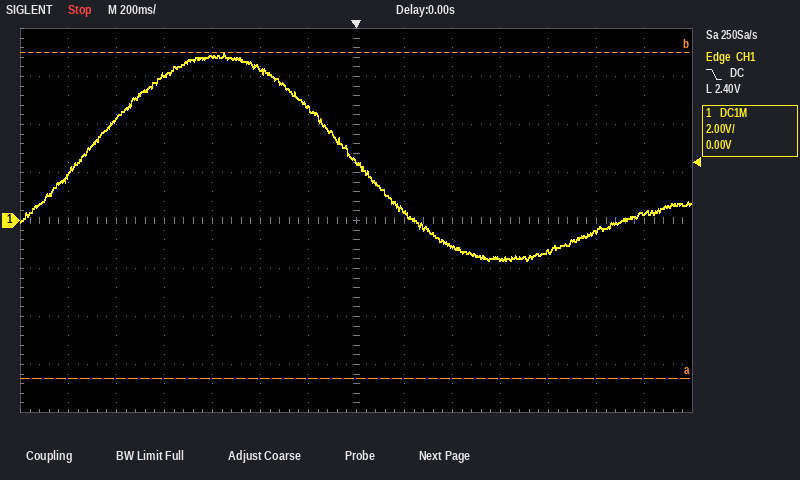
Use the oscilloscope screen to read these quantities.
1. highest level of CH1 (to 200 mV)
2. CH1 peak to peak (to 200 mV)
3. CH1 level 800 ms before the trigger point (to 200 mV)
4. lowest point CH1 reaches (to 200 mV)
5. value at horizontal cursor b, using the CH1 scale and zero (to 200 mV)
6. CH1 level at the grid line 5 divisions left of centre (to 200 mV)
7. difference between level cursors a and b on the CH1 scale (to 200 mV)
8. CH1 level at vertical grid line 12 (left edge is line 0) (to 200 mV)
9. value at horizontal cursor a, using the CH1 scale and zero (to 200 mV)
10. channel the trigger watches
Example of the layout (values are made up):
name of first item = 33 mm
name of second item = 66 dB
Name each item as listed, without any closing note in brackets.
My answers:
highest level of CH1 = 7.0 V
CH1 peak to peak = 8.6 V
CH1 level 800 ms before the trigger point = 6.0 V
lowest point CH1 reaches = -1.6 V
value at horizontal cursor b, using the CH1 scale and zero = 7.0 V
CH1 level at the grid line 5 divisions left of centre = 4.2 V
difference between level cursors a and b on the CH1 scale = 13.6 V
CH1 level at vertical grid line 12 (left edge is line 0) = -400 mV
value at horizontal cursor a, using the CH1 scale and zero = -6.6 V
channel the trigger watches = CH1
